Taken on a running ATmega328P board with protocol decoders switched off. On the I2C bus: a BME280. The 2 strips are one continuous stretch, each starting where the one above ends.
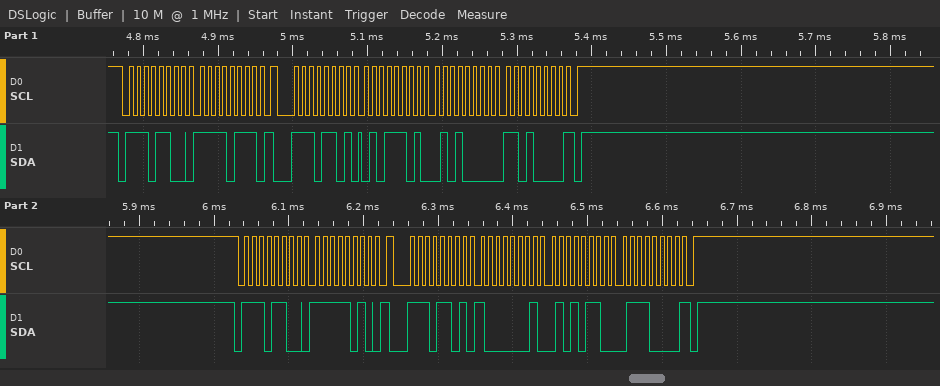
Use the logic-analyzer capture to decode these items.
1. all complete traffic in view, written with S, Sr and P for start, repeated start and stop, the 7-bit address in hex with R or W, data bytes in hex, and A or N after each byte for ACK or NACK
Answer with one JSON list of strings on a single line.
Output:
["S 76W A F7 A Sr 76R A 5D A 50 A D0 N P S 76W A FA A Sr 76R A 81 A 56 A 70 N P"]
